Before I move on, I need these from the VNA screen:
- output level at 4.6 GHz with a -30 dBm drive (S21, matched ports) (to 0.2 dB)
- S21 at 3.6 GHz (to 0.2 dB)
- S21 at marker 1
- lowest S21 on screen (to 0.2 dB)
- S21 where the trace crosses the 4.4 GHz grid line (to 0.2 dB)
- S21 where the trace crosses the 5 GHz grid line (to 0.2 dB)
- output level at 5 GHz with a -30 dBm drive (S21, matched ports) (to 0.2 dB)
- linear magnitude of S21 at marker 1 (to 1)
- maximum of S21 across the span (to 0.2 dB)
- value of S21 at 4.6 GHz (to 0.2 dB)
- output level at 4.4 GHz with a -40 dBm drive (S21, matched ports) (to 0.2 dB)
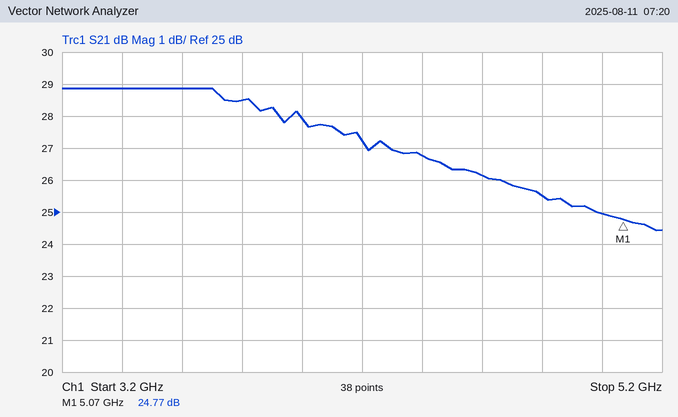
-3.8 dBm
28.8 dB
24.77 dB
24.4 dB
26.8 dB
25.0 dB
-5.0 dBm
17
28.8 dB
26.2 dB
-13.2 dBm
